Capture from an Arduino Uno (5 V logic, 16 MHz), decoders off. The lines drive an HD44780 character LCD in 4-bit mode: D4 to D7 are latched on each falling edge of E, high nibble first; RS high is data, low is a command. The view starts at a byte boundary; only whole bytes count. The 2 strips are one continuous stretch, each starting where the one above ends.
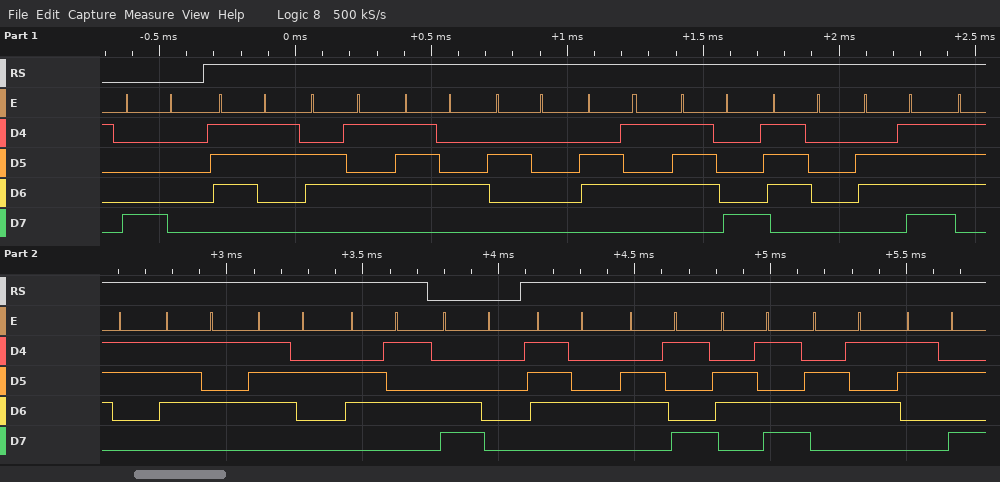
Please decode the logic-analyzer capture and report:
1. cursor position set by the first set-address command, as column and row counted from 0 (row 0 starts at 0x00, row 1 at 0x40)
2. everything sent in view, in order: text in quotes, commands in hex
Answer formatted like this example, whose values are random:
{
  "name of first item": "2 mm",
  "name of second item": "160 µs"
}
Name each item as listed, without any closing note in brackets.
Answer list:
{
  "cursor position set by the first set-address command, as column and row counted from 0": "column 0, row 0",
  "everything sent in view, in order: text in quotes, commands in hex": "0x80 \"set exposure\" 0xC0 \"time:\""
}
